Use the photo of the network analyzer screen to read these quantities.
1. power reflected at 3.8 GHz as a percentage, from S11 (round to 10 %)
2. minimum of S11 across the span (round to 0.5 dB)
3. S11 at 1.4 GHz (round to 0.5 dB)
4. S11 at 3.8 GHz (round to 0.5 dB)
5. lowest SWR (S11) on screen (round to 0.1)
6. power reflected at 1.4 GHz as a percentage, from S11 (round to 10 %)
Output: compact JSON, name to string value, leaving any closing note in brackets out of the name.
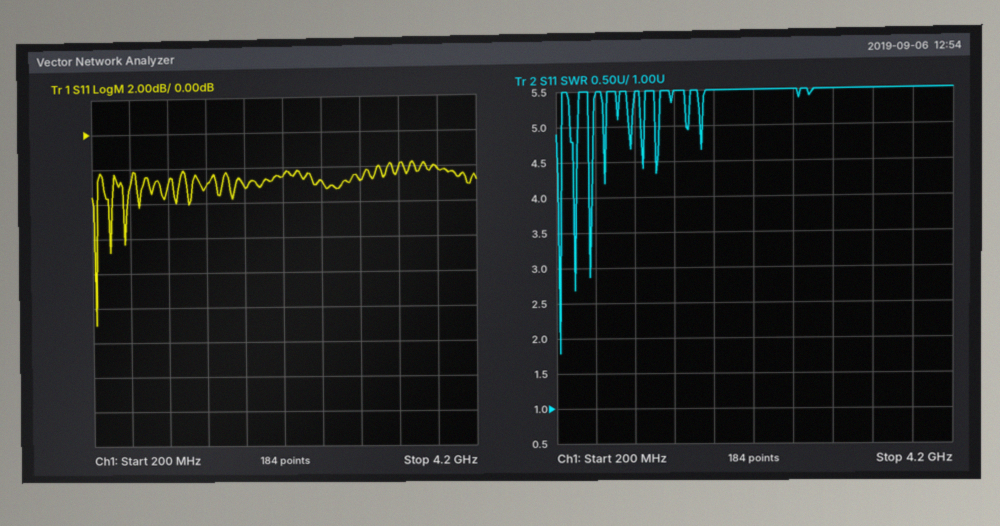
{"power reflected at 3.8 GHz as a percentage, from S11": "60 %", "minimum of S11 across the span": "-11.0 dB", "S11 at 1.4 GHz": "-3.0 dB", "S11 at 3.8 GHz": "-2.0 dB", "lowest SWR (S11) on screen": "1.8", "power reflected at 1.4 GHz as a percentage, from S11": "50 %"}
